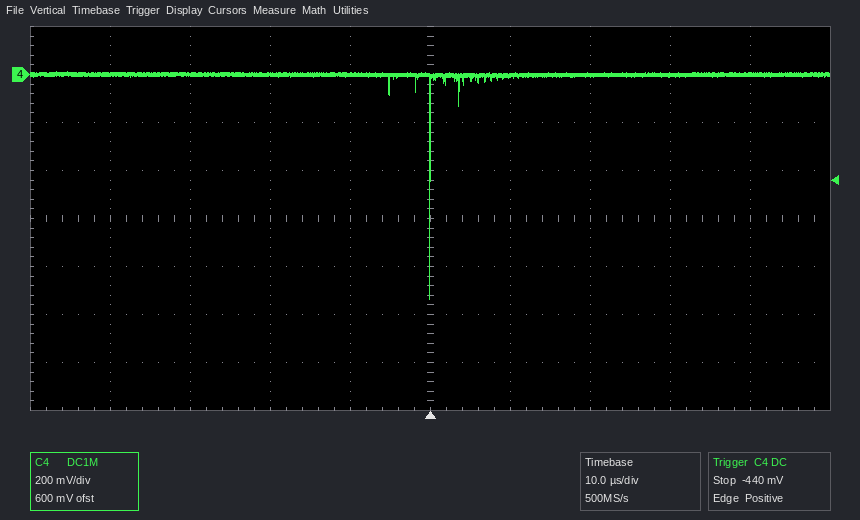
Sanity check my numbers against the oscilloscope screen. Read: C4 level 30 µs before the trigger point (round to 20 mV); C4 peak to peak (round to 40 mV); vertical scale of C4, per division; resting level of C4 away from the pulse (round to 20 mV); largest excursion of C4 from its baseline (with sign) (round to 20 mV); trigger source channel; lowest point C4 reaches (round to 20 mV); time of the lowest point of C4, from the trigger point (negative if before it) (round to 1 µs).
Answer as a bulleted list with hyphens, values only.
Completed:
- 0 mV
- 960 mV
- 200 mV
- 0 mV
- -940 mV
- C4
- -940 mV
- 0 µs
